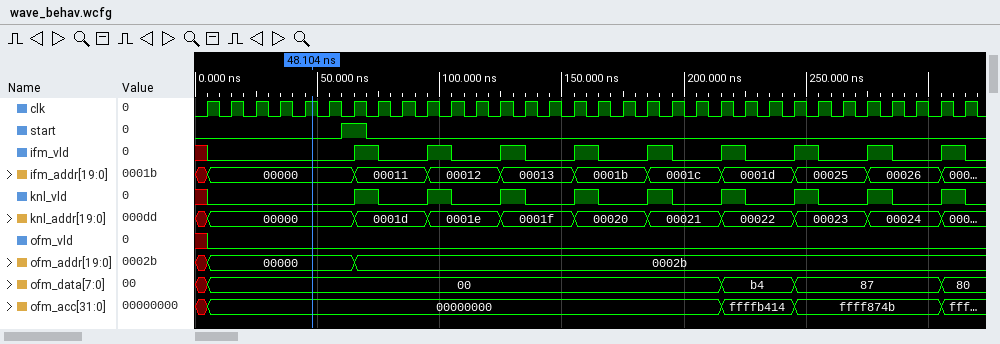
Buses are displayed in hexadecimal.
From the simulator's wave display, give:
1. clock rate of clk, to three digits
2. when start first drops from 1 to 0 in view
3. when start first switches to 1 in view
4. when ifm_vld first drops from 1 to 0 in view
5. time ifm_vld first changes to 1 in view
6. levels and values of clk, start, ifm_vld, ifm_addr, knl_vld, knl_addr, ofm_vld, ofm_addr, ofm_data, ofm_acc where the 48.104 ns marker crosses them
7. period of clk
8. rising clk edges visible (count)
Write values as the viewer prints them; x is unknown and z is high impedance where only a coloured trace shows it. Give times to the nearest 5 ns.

100 MHz
70 ns
60 ns
75 ns
65 ns
clk=1, start=0, ifm_vld=0, ifm_addr=00000, knl_vld=0, knl_addr=00000, ofm_vld=0, ofm_addr=00000, ofm_data=00, ofm_acc=00000000
10 ns
32
